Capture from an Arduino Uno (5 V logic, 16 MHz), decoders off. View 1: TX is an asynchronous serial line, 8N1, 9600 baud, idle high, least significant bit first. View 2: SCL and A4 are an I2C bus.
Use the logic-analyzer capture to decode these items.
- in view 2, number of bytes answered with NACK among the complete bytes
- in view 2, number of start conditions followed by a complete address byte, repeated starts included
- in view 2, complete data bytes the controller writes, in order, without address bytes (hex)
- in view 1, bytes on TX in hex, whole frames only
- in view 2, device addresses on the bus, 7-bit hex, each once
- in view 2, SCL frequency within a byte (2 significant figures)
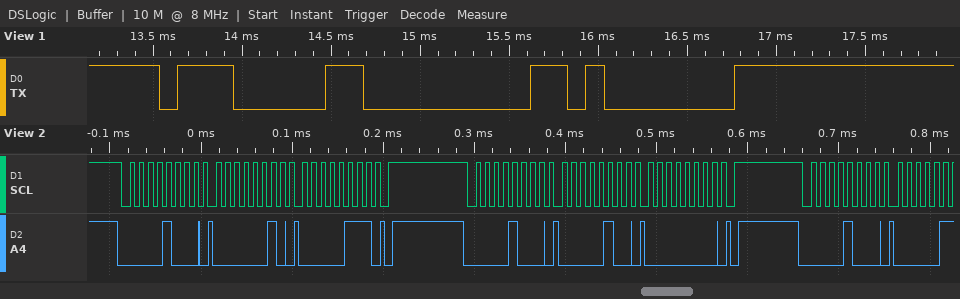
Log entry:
0
3
02 07 04 00
07 00 01
0x04
100 kHz
